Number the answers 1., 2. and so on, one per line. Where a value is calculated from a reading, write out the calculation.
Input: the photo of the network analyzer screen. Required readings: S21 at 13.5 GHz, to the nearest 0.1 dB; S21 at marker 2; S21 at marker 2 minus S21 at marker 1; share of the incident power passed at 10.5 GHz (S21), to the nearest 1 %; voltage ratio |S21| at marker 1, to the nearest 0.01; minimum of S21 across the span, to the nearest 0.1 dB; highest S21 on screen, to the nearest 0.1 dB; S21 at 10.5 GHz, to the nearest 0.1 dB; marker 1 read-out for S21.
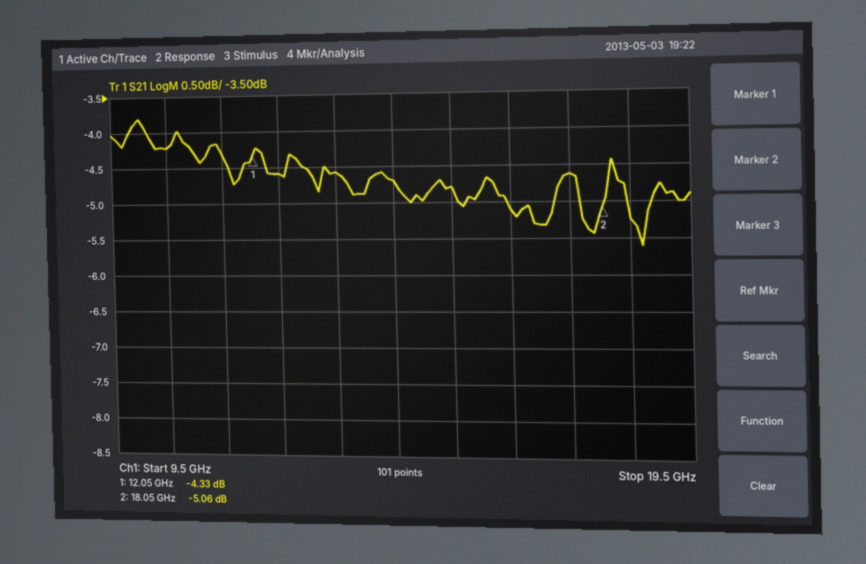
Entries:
1. -4.6 dB
2. -5.06 dB
3. -5.06 − (-4.33) = -0.73 dB
4. 10^(-4.2/10) ≈ 38 %
5. 10^(-4.33/20) ≈ 0.61
6. -5.6 dB
7. -3.8 dB
8. -4.2 dB
9. -4.33 dB
